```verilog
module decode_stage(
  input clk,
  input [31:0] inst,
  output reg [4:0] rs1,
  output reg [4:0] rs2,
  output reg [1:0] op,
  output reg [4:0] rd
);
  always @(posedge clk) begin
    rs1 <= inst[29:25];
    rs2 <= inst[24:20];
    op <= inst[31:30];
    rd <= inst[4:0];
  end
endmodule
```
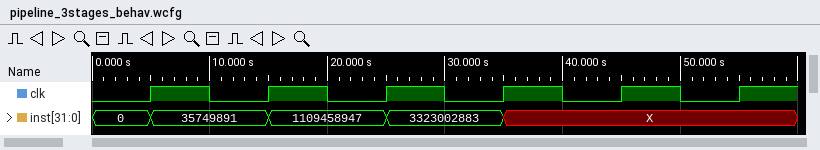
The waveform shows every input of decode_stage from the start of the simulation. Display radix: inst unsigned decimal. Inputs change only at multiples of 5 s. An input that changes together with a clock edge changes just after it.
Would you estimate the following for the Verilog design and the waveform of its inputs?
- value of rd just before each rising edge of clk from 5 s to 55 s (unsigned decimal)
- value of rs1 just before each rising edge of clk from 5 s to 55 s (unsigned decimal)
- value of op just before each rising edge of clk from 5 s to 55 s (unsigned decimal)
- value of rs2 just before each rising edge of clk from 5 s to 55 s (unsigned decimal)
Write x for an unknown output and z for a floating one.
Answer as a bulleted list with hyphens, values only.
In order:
- x, 0, 3, 3, 3, x
- x, 0, 1, 1, 3, x
- x, 0, 0, 1, 3, x
- x, 0, 2, 2, 1, x
